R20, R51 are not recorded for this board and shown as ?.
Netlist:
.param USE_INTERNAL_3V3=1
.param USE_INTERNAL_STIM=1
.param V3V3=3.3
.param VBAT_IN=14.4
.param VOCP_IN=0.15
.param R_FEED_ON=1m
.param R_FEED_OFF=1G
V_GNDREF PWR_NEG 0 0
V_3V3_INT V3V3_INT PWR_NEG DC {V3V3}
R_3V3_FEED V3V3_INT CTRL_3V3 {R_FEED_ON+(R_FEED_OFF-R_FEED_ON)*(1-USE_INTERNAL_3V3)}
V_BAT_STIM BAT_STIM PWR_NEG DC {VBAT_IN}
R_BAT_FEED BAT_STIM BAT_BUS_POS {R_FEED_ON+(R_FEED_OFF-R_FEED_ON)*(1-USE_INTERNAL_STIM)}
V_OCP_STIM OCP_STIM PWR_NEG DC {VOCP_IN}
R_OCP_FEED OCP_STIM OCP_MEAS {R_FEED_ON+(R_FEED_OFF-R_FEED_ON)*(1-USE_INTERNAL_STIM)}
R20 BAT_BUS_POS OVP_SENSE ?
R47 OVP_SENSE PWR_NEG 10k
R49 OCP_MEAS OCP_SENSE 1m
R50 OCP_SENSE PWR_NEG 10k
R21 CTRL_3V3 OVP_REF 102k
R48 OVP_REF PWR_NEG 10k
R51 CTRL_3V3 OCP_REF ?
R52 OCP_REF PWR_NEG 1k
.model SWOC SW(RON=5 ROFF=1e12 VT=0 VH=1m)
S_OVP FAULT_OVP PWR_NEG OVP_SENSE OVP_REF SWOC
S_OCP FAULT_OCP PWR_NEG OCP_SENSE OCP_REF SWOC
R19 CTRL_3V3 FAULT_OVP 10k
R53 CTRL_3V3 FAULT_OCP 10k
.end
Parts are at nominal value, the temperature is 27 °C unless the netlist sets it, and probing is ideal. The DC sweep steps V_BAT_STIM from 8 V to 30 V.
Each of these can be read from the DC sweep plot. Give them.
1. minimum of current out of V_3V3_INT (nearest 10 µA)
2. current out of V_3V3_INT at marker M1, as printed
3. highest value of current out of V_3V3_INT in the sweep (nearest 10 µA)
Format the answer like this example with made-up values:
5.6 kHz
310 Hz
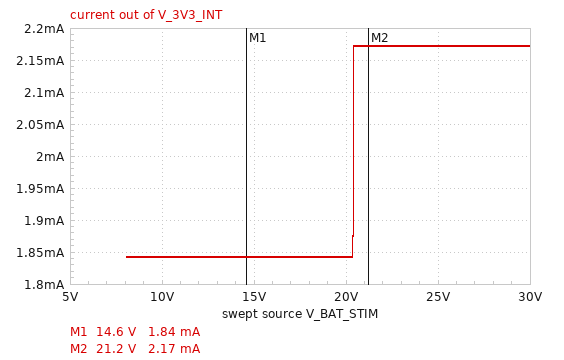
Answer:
1.84 mA
1.84 mA
2.17 mA
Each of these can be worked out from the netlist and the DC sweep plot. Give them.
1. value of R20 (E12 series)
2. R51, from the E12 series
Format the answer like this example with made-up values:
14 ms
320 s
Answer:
680 kΩ
820 Ω
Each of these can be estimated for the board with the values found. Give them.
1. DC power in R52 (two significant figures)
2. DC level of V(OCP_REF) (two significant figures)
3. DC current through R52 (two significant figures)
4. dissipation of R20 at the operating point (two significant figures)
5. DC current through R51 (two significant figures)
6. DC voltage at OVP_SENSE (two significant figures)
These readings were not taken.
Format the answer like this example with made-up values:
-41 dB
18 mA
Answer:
3.3 mW
1.8 V
1.8 mA
300 µW
1.8 mA
210 mV
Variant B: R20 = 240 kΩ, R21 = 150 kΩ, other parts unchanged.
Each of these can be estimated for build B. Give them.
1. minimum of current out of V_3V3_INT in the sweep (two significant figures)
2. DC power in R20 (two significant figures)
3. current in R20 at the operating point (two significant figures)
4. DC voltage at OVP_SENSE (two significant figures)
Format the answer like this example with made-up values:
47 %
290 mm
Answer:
2.2 mA
800 µW
58 µA
580 mV
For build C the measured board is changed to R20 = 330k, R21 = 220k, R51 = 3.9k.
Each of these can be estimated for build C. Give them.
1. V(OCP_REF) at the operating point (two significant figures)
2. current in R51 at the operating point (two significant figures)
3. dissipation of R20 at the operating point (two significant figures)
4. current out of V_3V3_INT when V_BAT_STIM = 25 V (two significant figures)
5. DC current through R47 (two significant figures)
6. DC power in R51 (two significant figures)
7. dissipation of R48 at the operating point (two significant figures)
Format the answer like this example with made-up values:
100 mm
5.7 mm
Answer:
670 mV
670 µA
590 µW
1.0 mA
42 µA
1.8 mW
2.1 µW
